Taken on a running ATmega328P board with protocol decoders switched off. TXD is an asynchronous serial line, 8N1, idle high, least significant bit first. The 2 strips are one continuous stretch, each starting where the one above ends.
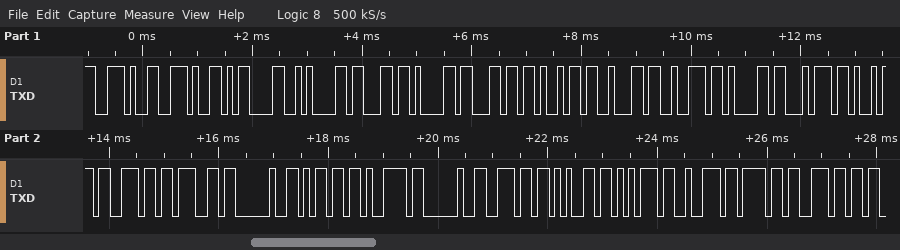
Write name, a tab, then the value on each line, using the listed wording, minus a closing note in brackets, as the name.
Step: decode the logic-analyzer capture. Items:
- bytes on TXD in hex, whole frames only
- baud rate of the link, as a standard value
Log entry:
bytes on TXD in hex, whole frames only	2E 2E 0D 0A 63 61 6C 69 62 72 61 74 69 6E 67 20 6D 79 20 6E 65 75 72 6F 6E
baud rate of the link, as a standard value	9600 baud
